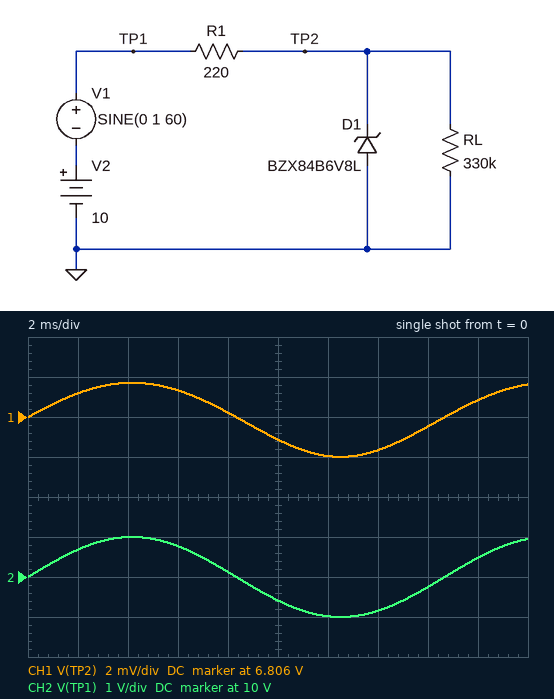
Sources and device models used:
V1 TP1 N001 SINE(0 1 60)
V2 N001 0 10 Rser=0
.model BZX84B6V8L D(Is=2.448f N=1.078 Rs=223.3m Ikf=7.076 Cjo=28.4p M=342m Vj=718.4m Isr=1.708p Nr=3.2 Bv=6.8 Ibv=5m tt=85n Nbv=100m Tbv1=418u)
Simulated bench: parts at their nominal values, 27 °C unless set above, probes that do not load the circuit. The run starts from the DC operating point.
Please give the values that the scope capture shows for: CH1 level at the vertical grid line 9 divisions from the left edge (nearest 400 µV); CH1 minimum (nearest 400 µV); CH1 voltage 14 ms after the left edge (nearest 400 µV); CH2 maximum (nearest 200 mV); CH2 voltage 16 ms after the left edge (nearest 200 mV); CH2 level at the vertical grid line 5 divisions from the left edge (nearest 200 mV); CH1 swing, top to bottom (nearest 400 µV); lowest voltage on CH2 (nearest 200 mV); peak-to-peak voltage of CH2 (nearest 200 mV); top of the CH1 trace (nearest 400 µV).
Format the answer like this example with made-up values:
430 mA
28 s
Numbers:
6.8068 V
6.8040 V
6.8044 V
11.0 V
9.8 V
9.4 V
3.6 mV
9.0 V
2.0 V
6.8076 V
